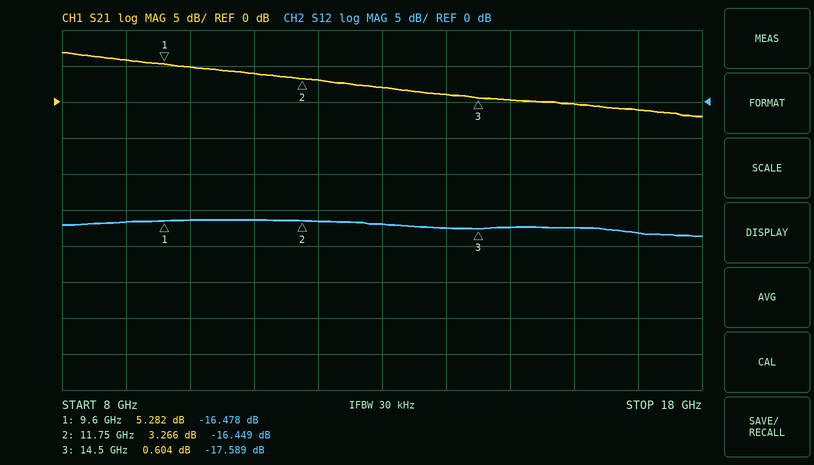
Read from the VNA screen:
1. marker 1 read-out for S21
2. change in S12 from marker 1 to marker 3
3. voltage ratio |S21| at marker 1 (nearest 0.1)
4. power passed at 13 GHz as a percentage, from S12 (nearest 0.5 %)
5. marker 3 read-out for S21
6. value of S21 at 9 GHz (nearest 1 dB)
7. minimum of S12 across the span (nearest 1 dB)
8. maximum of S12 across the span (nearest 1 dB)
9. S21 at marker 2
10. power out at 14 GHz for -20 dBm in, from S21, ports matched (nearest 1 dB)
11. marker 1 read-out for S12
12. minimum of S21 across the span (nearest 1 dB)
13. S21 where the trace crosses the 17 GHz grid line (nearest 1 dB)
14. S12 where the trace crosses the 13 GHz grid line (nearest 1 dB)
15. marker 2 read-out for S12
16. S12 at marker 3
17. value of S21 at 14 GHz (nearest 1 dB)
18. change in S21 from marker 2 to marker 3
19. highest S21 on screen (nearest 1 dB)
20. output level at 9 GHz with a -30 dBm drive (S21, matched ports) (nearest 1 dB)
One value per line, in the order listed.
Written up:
5.282 dB
-1.111 dB
1.8
2.0 %
0.604 dB
6 dB
-19 dB
-16 dB
3.266 dB
-19 dBm
-16.478 dB
-2 dB
-1 dB
-17 dB
-16.449 dB
-17.589 dB
1 dB
-2.662 dB
7 dB
-24 dBm
